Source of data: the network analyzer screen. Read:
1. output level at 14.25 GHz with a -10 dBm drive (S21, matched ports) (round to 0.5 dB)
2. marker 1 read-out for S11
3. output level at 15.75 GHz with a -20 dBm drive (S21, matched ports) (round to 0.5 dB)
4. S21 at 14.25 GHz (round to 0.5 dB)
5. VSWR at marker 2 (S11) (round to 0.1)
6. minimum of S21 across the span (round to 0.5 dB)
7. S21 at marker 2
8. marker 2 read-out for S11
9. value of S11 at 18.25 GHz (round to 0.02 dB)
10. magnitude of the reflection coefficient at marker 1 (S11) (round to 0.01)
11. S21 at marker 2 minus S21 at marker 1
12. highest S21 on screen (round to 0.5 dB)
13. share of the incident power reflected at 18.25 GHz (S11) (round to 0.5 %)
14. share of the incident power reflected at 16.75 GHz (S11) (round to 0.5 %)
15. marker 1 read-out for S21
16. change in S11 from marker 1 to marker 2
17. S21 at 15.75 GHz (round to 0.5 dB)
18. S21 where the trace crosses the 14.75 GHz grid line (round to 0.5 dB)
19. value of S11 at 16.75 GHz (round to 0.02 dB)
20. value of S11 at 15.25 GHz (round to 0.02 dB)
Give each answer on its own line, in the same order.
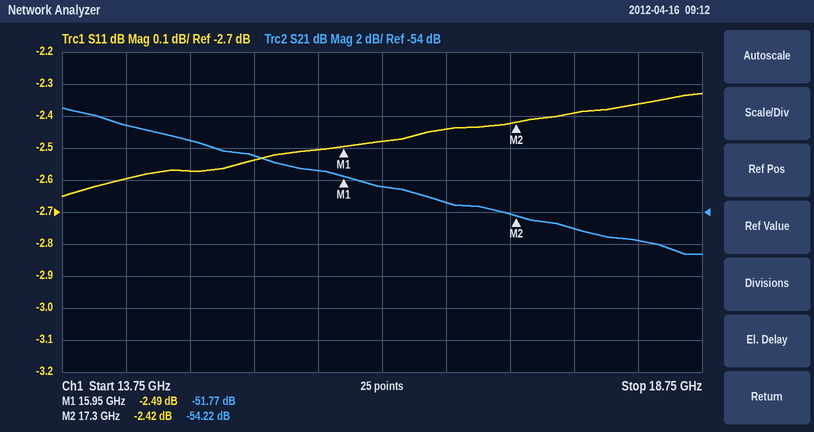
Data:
-58.5 dBm
-2.49 dB
-71.5 dBm
-48.5 dB
7.2
-56.5 dB
-54.22 dB
-2.42 dB
-2.36 dB
0.75
-2.45 dB
-47.5 dB
58.0 %
57.0 %
-51.77 dB
0.07 dB
-51.5 dB
-49.5 dB
-2.44 dB
-2.54 dB
